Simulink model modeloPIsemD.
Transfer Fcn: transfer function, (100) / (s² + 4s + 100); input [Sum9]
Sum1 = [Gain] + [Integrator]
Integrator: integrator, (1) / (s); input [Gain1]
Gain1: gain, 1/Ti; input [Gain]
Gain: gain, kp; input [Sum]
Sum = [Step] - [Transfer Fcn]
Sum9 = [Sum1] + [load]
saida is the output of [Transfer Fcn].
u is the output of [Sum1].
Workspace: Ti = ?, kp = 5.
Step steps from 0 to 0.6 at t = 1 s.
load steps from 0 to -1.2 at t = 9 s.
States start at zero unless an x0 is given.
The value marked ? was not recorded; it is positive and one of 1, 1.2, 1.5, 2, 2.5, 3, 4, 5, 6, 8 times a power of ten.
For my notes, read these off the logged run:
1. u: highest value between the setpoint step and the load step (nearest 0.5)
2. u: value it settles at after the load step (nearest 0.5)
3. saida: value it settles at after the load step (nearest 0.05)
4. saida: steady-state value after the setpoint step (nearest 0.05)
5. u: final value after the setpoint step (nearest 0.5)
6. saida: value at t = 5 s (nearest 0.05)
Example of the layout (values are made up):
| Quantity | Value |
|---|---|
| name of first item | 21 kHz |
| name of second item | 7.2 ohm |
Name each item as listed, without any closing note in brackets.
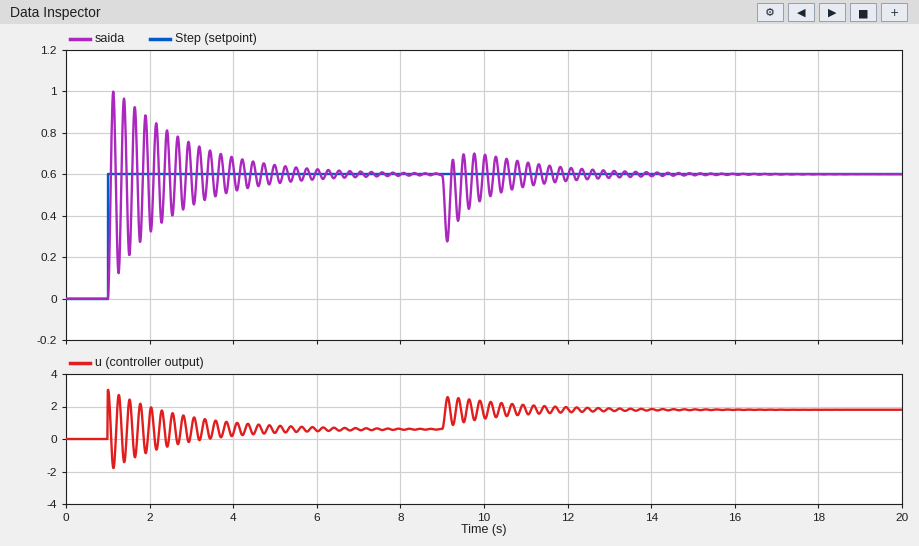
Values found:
| Quantity | Value |
|---|---|
| u: highest value between the setpoint step and the load step | 3.0 |
| u: value it settles at after the load step | 2.0 |
| saida: value it settles at after the load step | 0.60 |
| saida: steady-state value after the setpoint step | 0.60 |
| u: final value after the setpoint step | 0.5 |
| saida: value at t = 5 s | 0.65 |
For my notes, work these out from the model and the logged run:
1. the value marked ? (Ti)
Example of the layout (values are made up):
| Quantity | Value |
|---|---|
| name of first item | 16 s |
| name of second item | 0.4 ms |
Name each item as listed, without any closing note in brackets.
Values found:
| Quantity | Value |
|---|---|
| the value marked ? | 0.3 |
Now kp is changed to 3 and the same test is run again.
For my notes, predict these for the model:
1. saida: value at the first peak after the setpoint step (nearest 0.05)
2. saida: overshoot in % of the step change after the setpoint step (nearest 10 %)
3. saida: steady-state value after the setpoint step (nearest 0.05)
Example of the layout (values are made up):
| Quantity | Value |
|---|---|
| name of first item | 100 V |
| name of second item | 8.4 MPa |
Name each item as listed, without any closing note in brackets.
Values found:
| Quantity | Value |
|---|---|
| saida: value at the first peak after the setpoint step | 0.90 |
| saida: overshoot in % of the step change after the setpoint step | 50 % |
| saida: steady-state value after the setpoint step | 0.60 |
